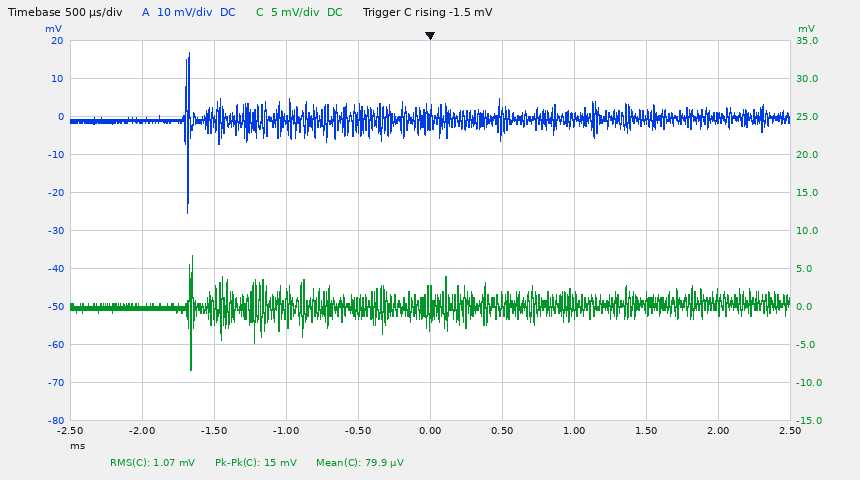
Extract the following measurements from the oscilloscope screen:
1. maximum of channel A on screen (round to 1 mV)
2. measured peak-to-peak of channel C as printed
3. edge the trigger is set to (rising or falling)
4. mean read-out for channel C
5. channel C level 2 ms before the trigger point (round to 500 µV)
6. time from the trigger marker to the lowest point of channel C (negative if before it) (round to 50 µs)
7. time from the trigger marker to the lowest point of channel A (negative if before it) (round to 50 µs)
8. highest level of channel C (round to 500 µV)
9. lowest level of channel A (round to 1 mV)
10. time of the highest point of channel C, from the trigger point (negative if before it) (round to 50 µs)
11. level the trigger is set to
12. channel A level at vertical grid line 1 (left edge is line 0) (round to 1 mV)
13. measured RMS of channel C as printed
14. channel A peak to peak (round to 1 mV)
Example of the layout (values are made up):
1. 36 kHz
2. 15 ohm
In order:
1. 17 mV
2. 15 mV
3. rising
4. 79.9 µV
5. 0.0 mV
6. -1.65 ms
7. -1.70 ms
8. 6.5 mV
9. -25 mV
10. -1.65 ms
11. -1.5 mV
12. -1 mV
13. 1.07 mV
14. 42 mV
